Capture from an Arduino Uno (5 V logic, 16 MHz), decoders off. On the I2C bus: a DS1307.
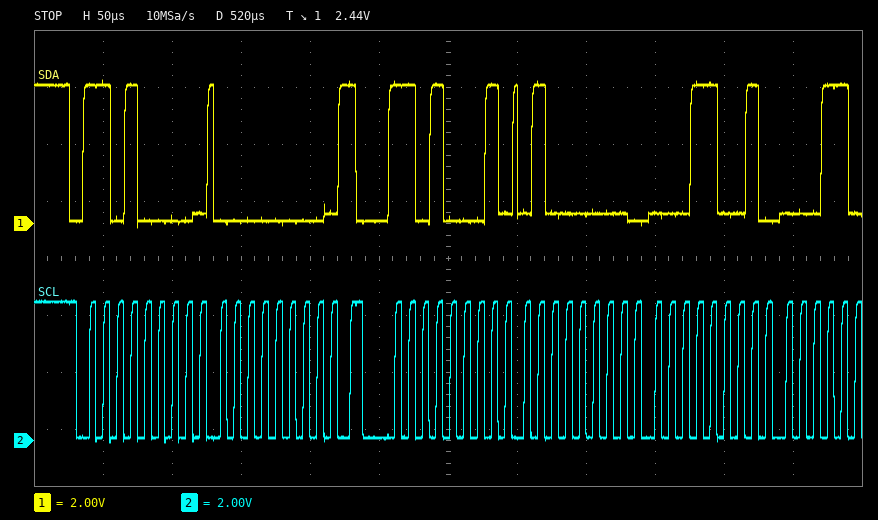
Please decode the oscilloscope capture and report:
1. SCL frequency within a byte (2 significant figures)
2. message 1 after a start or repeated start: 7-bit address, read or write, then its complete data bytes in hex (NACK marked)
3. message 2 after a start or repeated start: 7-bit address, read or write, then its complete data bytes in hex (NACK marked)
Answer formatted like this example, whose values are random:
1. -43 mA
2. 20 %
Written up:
1. 100 kHz
2. 0x68 write: 00
3. 0x68 read: 40 19
